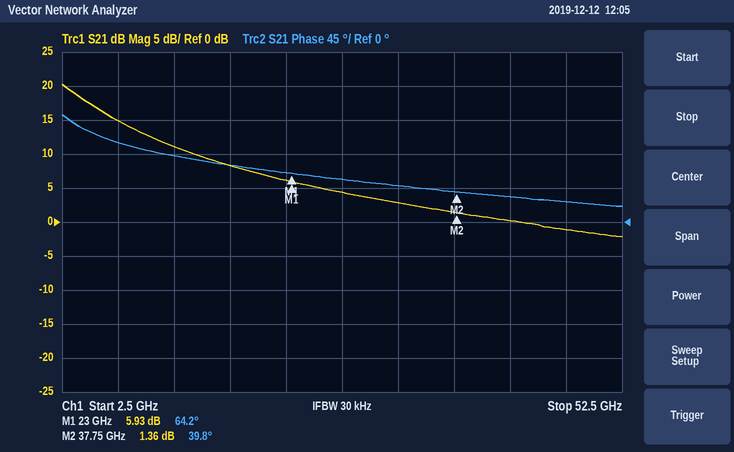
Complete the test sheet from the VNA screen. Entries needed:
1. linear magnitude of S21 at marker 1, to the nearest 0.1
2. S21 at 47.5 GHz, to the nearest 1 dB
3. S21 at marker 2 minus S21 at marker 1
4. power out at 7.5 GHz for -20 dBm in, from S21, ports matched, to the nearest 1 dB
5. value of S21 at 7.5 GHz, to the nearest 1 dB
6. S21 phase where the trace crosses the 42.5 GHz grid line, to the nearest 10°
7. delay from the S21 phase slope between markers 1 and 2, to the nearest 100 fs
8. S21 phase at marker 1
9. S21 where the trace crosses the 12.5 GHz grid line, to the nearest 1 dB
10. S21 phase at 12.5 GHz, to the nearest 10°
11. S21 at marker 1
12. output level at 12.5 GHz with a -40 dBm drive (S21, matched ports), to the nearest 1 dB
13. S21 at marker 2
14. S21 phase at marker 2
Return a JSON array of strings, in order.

["2.0", "-1 dB", "-4.57 dB", "-5 dBm", "15 dB", "30°", "4.6 ps", "64.2°", "11 dB", "90°", "5.93 dB", "-29 dBm", "1.36 dB", "39.8°"]
